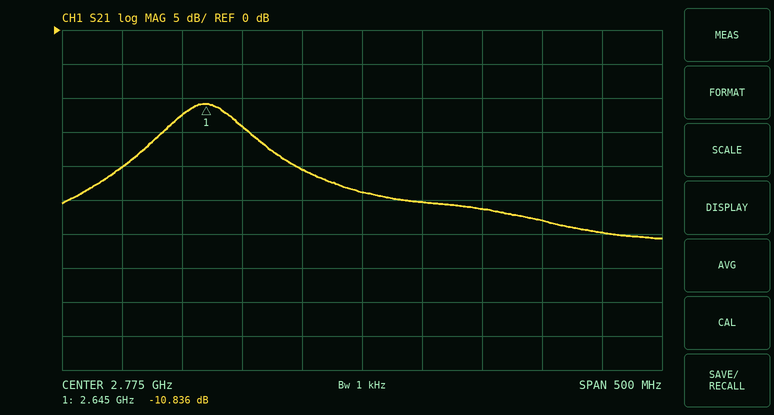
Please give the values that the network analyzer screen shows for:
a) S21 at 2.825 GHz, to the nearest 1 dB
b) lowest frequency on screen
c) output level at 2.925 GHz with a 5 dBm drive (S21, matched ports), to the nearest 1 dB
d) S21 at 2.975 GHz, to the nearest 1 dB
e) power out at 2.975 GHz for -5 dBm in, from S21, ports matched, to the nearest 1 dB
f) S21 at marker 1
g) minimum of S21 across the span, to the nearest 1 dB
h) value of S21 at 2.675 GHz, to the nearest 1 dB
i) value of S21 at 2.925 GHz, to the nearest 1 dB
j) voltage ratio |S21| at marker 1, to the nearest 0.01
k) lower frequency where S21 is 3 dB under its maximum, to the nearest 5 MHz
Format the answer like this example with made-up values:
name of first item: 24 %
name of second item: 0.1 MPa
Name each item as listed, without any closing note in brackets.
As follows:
S21 at 2.825 GHz, to the nearest 1 dB: -25 dB
lowest frequency on screen: 2.525 GHz
output level at 2.925 GHz with a 5 dBm drive (S21, matched ports), to the nearest 1 dB: -23 dBm
S21 at 2.975 GHz, to the nearest 1 dB: -30 dB
power out at 2.975 GHz for -5 dBm in, from S21, ports matched, to the nearest 1 dB: -35 dBm
S21 at marker 1: -10.836 dB
minimum of S21 across the span, to the nearest 1 dB: -31 dB
value of S21 at 2.675 GHz, to the nearest 1 dB: -14 dB
value of S21 at 2.925 GHz, to the nearest 1 dB: -28 dB
voltage ratio |S21| at marker 1, to the nearest 0.01: 0.29
lower frequency where S21 is 3 dB under its maximum, to the nearest 5 MHz: 2.615 GHz
